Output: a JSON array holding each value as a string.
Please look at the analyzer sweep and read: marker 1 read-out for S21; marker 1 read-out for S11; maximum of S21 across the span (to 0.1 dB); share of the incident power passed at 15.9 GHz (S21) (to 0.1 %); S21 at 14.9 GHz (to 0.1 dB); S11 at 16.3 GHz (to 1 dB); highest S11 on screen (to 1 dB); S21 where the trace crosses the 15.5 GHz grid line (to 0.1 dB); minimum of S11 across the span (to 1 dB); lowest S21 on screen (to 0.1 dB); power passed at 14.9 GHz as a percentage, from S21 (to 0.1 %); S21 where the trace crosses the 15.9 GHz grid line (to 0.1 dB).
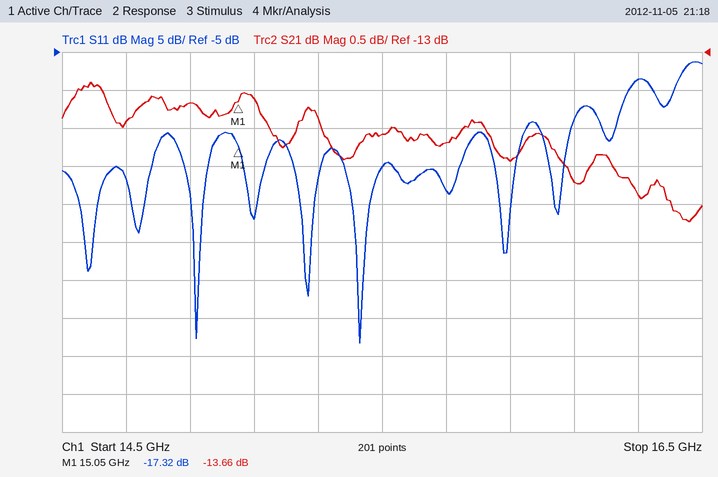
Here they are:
["-13.66 dB", "-17.32 dB", "-13.4 dB", "3.6 %", "-13.7 dB", "-9 dB", "-6 dB", "-14.1 dB", "-43 dB", "-15.2 dB", "4.3 %", "-14.4 dB"]
